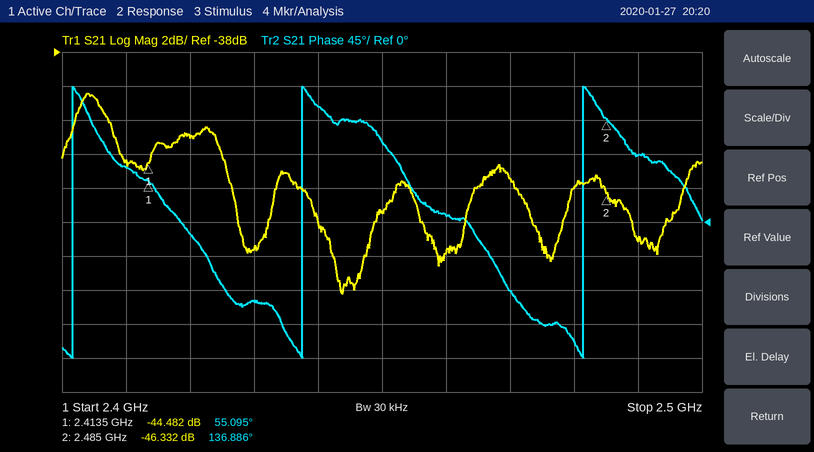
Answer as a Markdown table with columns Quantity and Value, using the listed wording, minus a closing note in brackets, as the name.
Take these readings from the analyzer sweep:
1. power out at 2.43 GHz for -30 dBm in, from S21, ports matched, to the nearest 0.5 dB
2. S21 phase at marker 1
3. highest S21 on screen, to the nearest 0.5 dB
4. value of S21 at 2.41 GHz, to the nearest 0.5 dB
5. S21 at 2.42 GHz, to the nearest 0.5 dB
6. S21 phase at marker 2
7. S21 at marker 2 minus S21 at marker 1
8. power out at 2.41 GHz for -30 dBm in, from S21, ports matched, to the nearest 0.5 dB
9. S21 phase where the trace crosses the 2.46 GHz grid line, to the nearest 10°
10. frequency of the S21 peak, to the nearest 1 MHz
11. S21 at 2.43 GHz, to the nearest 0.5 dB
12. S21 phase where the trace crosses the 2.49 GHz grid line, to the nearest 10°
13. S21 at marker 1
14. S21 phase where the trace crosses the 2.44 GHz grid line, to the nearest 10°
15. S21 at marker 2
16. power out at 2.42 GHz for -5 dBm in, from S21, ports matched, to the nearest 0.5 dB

| Quantity | Value |
|---|---|
| power out at 2.43 GHz for -30 dBm in, from S21, ports matched, to the nearest 0.5 dB | -79.5 dBm |
| S21 phase at marker 1 | 55.095° |
| highest S21 on screen, to the nearest 0.5 dB | -40.5 dB |
| value of S21 at 2.41 GHz, to the nearest 0.5 dB | -44.5 dB |
| S21 at 2.42 GHz, to the nearest 0.5 dB | -43.0 dB |
| S21 phase at marker 2 | 136.886° |
| S21 at marker 2 minus S21 at marker 1 | -1.850 dB |
| power out at 2.41 GHz for -30 dBm in, from S21, ports matched, to the nearest 0.5 dB | -74.5 dBm |
| S21 phase where the trace crosses the 2.46 GHz grid line, to the nearest 10° | 10° |
| frequency of the S21 peak, to the nearest 1 MHz | 2.404 GHz |
| S21 at 2.43 GHz, to the nearest 0.5 dB | -49.5 dB |
| S21 phase where the trace crosses the 2.49 GHz grid line, to the nearest 10° | 90° |
| S21 at marker 1 | -44.482 dB |
| S21 phase where the trace crosses the 2.44 GHz grid line, to the nearest 10° | 150° |
| S21 at marker 2 | -46.332 dB |
| power out at 2.42 GHz for -5 dBm in, from S21, ports matched, to the nearest 0.5 dB | -48.0 dBm |
